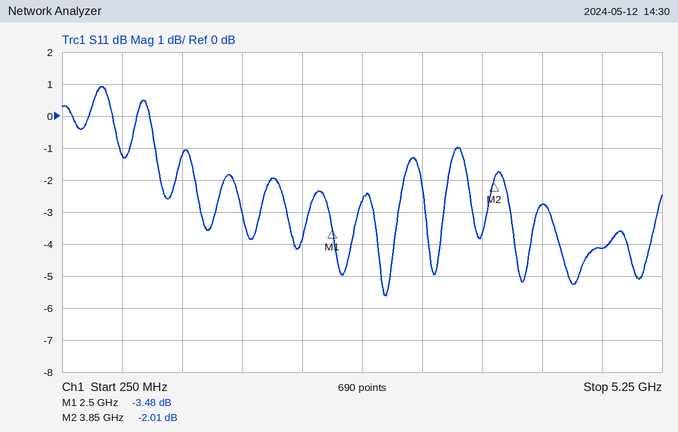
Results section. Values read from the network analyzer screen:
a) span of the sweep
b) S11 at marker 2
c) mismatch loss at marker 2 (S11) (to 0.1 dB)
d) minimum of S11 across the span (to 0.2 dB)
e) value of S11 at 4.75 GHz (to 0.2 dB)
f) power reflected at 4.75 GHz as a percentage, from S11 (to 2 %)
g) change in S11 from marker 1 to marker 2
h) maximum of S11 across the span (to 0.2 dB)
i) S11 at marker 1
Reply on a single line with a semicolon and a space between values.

5 GHz; -2.01 dB; 4.3 dB; -5.6 dB; -4.2 dB; 38 %; 1.47 dB; 1.0 dB; -3.48 dB
